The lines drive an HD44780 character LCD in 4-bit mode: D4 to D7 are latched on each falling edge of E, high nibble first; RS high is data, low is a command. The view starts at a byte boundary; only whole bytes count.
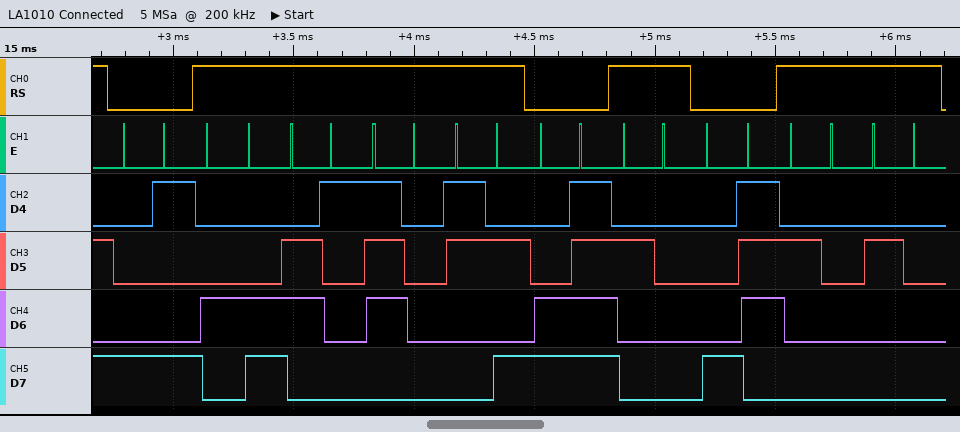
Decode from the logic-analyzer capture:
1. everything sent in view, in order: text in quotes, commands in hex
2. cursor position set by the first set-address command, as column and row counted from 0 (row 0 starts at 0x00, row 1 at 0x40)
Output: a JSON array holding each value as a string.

["0x89 \"Lap:\" 0xCF \" \" 0x87 \"  \"", "column 9, row 0"]
